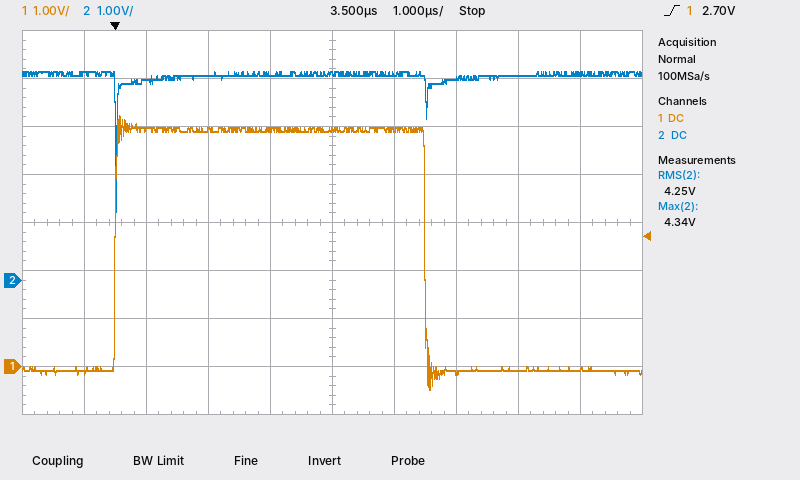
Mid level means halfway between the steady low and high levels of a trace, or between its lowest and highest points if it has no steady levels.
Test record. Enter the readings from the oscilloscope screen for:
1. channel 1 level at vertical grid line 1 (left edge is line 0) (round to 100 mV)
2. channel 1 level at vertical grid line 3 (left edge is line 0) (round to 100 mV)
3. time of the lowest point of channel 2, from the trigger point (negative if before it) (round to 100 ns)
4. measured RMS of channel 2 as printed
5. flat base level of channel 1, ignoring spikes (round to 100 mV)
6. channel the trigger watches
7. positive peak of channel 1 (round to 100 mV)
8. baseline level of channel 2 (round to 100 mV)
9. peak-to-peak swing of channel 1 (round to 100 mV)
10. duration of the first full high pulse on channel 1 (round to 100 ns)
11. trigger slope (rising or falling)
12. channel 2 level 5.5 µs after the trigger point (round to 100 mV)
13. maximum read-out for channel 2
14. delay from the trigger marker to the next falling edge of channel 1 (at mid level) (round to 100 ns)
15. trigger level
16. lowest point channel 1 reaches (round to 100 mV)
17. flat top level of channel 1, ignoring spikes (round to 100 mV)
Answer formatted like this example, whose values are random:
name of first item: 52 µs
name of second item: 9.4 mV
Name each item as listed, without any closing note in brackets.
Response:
channel 1 level at vertical grid line 1 (left edge is line 0): -100 mV
channel 1 level at vertical grid line 3 (left edge is line 0): 4.9 V
time of the lowest point of channel 2, from the trigger point (negative if before it): 0.0 µs
measured RMS of channel 2 as printed: 4.25 V
flat base level of channel 1, ignoring spikes: -100 mV
channel the trigger watches: channel 1
positive peak of channel 1: 5.2 V
baseline level of channel 2: 4.3 V
peak-to-peak swing of channel 1: 5.7 V
duration of the first full high pulse on channel 1: 5.0 µs
trigger slope: rising
channel 2 level 5.5 µs after the trigger point: 4.2 V
maximum read-out for channel 2: 4.34 V
delay from the trigger marker to the next falling edge of channel 1 (at mid level): 5.0 µs
trigger level: 2.70 V
lowest point channel 1 reaches: -500 mV
flat top level of channel 1, ignoring spikes: 4.9 V
